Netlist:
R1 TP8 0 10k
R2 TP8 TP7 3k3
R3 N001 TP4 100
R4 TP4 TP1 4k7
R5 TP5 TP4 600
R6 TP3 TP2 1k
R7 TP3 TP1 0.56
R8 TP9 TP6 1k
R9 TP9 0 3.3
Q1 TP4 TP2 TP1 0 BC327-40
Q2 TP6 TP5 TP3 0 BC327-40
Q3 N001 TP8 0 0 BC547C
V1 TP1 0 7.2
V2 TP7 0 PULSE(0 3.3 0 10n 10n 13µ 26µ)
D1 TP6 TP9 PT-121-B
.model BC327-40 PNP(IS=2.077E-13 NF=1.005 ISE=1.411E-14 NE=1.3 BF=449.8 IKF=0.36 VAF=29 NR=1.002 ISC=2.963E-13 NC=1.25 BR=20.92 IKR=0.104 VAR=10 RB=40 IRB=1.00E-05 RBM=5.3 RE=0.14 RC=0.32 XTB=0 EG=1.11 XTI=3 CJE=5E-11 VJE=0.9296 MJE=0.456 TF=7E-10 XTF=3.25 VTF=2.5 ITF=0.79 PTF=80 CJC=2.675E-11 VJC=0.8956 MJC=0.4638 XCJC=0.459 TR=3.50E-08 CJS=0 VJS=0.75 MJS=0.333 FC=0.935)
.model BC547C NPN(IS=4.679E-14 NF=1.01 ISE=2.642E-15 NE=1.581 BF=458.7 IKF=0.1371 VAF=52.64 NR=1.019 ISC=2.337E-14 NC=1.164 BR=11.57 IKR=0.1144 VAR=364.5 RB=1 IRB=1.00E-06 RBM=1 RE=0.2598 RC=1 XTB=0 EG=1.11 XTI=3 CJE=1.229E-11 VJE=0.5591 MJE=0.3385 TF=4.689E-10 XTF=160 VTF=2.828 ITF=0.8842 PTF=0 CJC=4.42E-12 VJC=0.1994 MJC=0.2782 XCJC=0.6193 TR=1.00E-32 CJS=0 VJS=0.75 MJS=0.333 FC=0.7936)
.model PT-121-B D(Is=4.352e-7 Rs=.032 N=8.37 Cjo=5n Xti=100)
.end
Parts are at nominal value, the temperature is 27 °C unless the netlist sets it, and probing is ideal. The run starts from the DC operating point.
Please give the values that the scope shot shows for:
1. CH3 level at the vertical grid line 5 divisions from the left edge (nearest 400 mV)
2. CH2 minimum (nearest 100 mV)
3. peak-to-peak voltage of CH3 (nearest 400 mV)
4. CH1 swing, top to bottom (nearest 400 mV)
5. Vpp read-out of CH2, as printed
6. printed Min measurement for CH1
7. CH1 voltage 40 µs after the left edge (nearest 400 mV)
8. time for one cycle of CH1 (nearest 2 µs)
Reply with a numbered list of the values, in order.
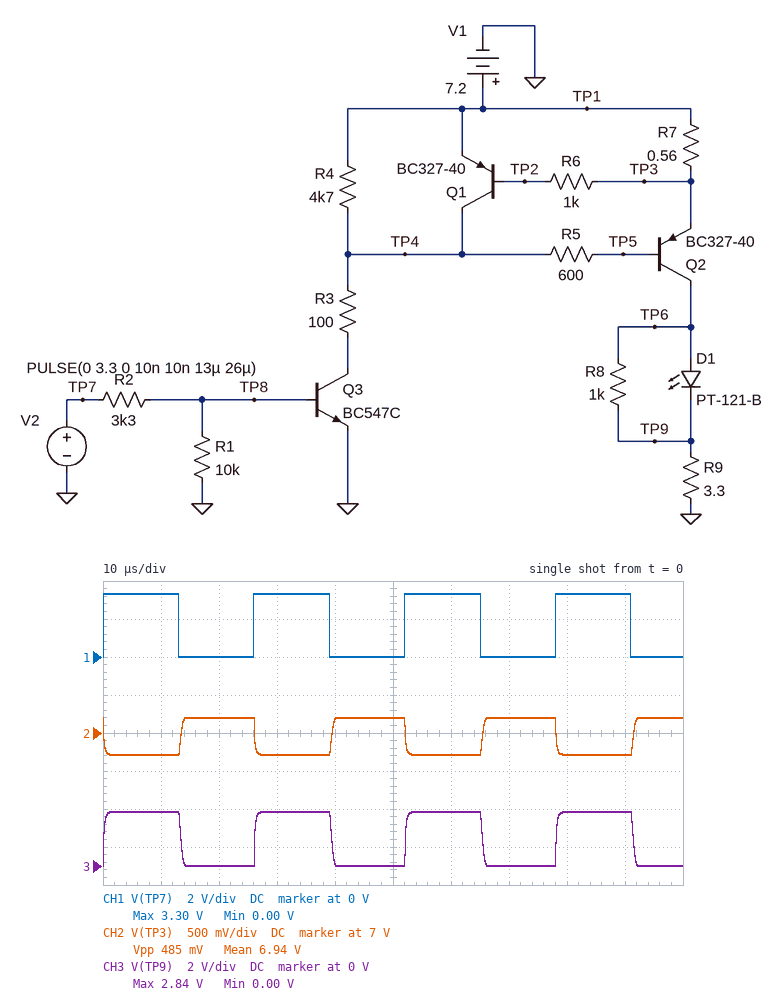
1. 0 V
2. 6.7 V
3. 2.8 V
4. 3.2 V
5. 485 mV
6. 0.00 V
7. 0 V
8. 26 µs
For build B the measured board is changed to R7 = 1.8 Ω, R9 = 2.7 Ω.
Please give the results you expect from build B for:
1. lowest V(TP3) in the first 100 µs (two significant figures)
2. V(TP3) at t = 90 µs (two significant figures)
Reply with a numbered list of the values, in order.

1. 6.2 V
2. 6.4 V
